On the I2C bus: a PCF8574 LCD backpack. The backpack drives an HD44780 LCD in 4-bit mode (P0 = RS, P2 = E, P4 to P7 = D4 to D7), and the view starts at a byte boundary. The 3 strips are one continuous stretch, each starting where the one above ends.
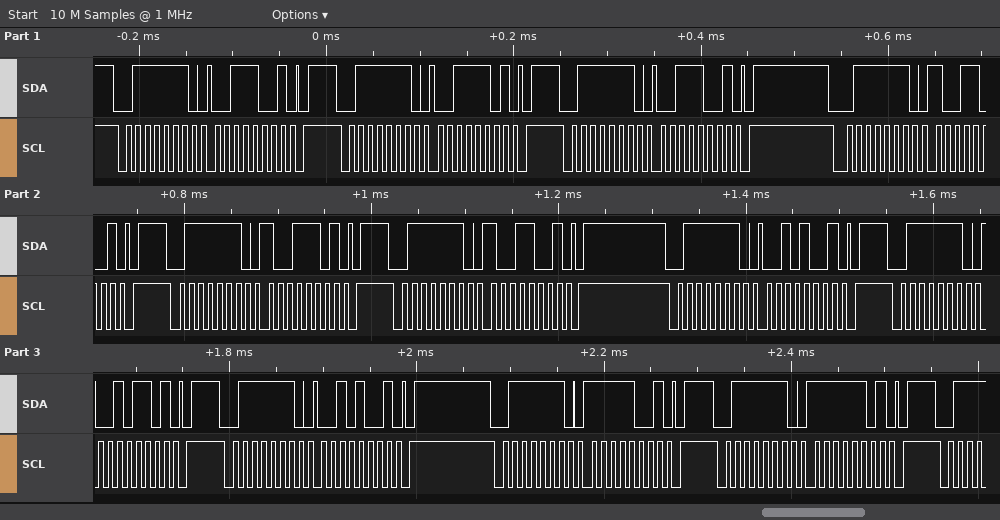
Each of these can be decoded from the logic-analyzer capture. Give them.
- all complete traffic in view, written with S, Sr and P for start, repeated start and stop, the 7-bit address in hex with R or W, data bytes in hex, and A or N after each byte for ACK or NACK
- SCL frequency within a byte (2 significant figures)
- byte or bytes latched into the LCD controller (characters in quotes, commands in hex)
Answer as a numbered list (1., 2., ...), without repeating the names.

1. S 3FW A 39 A P S 3FW A 3D A P S 3FW A 39 A P S 3FW A 99 A P S 3FW A 9D A P S 3FW A 99 A P S 3FW A 29 A P S 3FW A 2D A P S 3FW A 29 A P S 3FW A F9 A P S 3FW A FD A P
2. 100 kHz
3. '9'
